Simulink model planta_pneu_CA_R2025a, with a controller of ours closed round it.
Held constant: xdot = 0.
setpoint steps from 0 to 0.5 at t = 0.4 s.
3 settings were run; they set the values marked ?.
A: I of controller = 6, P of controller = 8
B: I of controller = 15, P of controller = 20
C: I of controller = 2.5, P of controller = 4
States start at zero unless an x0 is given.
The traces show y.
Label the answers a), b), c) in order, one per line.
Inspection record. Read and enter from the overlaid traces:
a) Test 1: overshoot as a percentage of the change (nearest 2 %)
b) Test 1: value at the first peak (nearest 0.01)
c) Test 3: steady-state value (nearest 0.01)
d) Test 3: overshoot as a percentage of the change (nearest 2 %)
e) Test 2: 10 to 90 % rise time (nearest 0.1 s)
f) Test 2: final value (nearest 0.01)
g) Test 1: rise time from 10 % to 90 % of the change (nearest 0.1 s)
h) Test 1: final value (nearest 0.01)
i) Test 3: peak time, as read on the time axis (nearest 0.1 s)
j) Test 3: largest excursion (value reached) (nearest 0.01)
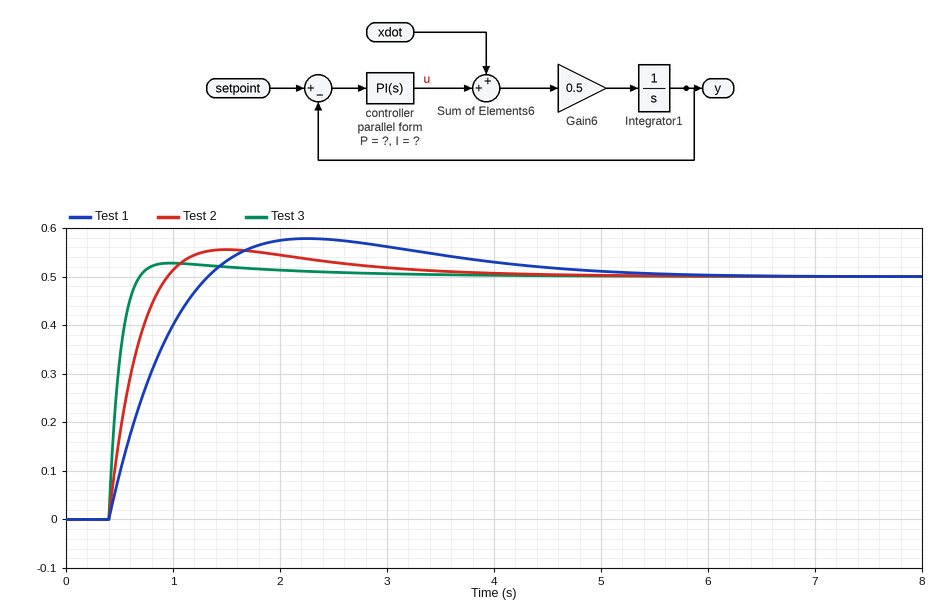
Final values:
a) 16 %
b) 0.58
c) 0.50
d) 6 %
e) 0.4 s
f) 0.50
g) 0.7 s
h) 0.50
i) 1.0 s
j) 0.53
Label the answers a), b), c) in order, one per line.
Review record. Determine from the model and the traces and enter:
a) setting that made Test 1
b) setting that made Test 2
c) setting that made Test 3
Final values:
a) C
b) A
c) B
